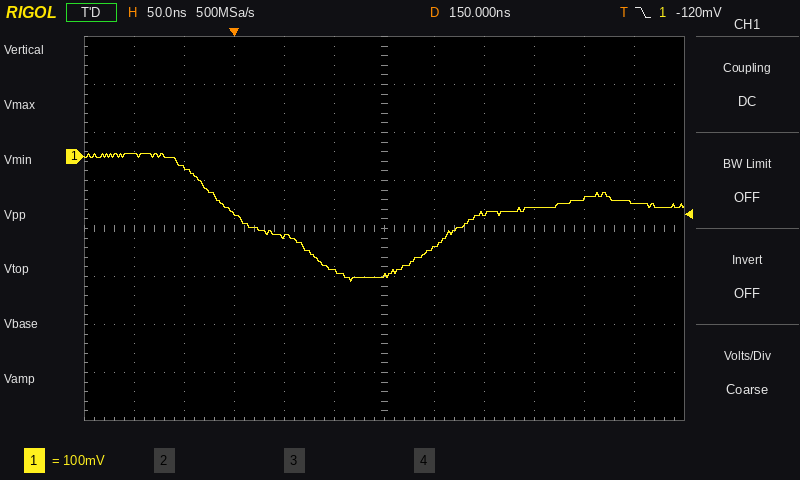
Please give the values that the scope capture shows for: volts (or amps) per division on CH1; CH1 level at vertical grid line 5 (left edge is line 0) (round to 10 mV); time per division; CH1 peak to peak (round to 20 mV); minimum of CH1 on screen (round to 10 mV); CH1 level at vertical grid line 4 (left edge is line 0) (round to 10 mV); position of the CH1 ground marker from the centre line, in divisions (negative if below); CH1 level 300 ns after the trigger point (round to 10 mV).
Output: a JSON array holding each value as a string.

["100 mV", "-240 mV", "50 ns", "260 mV", "-260 mV", "-170 mV", "+1.5 div", "-110 mV"]
